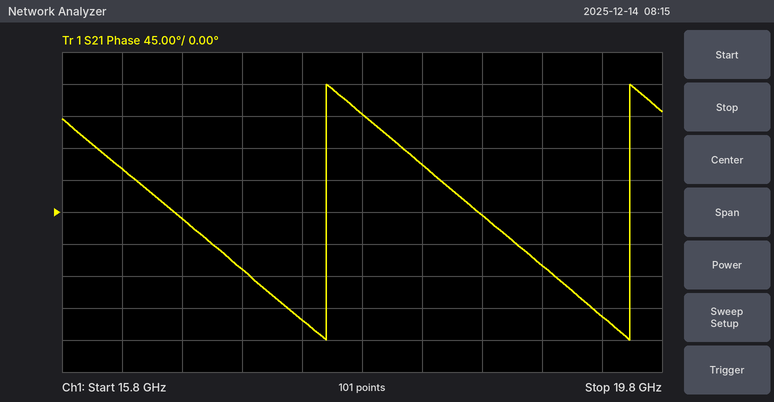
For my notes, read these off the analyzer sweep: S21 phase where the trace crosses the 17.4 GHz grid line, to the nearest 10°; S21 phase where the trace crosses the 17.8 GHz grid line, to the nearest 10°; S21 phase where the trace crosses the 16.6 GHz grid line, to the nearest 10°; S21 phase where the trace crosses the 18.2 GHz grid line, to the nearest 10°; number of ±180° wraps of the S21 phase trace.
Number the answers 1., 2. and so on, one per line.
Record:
1. -150°
2. 140°
3. -10°
4. 70°
5. 2
